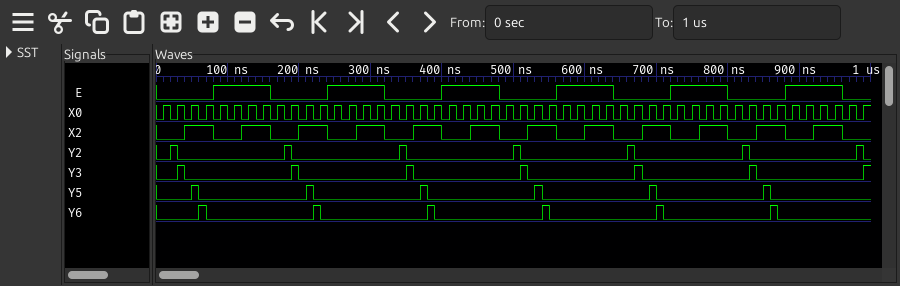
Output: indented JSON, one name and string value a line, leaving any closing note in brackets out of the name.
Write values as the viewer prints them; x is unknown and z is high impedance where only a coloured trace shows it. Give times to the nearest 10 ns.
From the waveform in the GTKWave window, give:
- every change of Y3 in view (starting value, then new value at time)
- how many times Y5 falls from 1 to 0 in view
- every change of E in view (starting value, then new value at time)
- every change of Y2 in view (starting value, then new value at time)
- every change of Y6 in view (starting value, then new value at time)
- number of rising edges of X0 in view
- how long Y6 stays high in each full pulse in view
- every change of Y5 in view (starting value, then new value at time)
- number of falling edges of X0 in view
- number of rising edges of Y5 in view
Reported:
{
  "every change of Y3 in view": "0, 1 at 30 ns, 0 at 40 ns, 1 at 190 ns, 0 at 200 ns, 1 at 350 ns, 0 at 360 ns, 1 at 510 ns, 0 at 520 ns, 1 at 670 ns, 0 at 680 ns, 1 at 830 ns, 0 at 840 ns, 1 at 990 ns",
  "how many times Y5 falls from 1 to 0 in view": "6",
  "every change of E in view": "0, 1 at 80 ns, 0 at 160 ns, 1 at 240 ns, 0 at 320 ns, 1 at 400 ns, 0 at 480 ns, 1 at 560 ns, 0 at 640 ns, 1 at 720 ns, 0 at 800 ns, 1 at 880 ns, 0 at 960 ns",
  "every change of Y2 in view": "0, 1 at 20 ns, 0 at 30 ns, 1 at 180 ns, 0 at 190 ns, 1 at 340 ns, 0 at 350 ns, 1 at 500 ns, 0 at 510 ns, 1 at 660 ns, 0 at 670 ns, 1 at 820 ns, 0 at 830 ns, 1 at 980 ns, 0 at 990 ns",
  "every change of Y6 in view": "0, 1 at 60 ns, 0 at 70 ns, 1 at 220 ns, 0 at 230 ns, 1 at 380 ns, 0 at 390 ns, 1 at 540 ns, 0 at 550 ns, 1 at 700 ns, 0 at 710 ns, 1 at 860 ns, 0 at 870 ns",
  "number of rising edges of X0 in view": "50",
  "how long Y6 stays high in each full pulse in view": "10 ns, 10 ns, 10 ns, 10 ns, 10 ns, 10 ns",
  "every change of Y5 in view": "0, 1 at 50 ns, 0 at 60 ns, 1 at 210 ns, 0 at 220 ns, 1 at 370 ns, 0 at 380 ns, 1 at 530 ns, 0 at 540 ns, 1 at 690 ns, 0 at 700 ns, 1 at 850 ns, 0 at 860 ns",
  "number of falling edges of X0 in view": "49",
  "number of rising edges of Y5 in view": "6"
}
